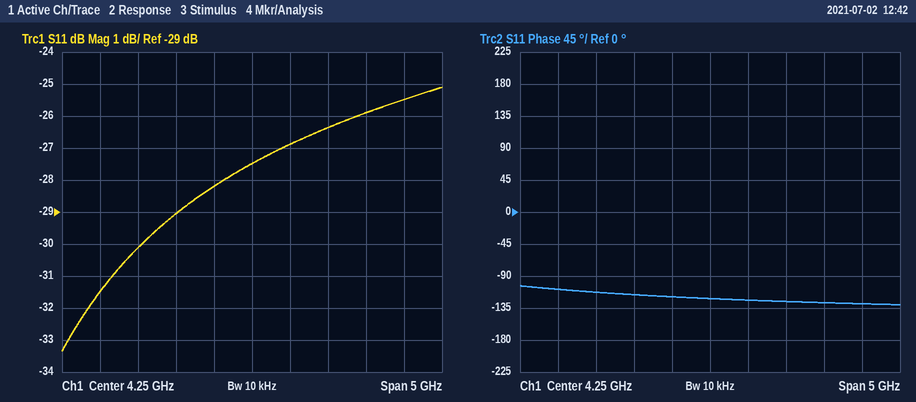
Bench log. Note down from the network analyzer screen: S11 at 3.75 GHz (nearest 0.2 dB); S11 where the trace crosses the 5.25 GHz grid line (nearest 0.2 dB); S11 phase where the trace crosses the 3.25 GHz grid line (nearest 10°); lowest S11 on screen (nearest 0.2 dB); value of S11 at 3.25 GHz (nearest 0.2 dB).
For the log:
-28.2 dB
-26.4 dB
-120°
-33.4 dB
-29.0 dB
